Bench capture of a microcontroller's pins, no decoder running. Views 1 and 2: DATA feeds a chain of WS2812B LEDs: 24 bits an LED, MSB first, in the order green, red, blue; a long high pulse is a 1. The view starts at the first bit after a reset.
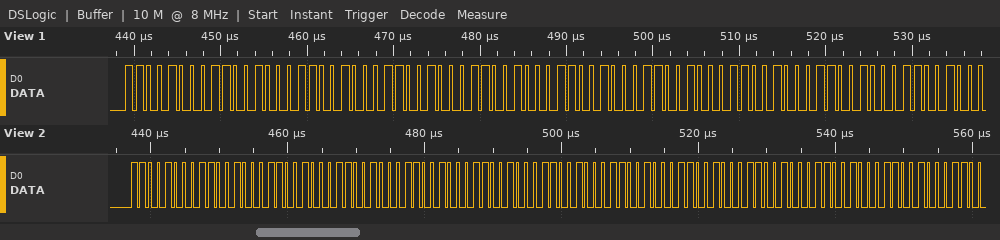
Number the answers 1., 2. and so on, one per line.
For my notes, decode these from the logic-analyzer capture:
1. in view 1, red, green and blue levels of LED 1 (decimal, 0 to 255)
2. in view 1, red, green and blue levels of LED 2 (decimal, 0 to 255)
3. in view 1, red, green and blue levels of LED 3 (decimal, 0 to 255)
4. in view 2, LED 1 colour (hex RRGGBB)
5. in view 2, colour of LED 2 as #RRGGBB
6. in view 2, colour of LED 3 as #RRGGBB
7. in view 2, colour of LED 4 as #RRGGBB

1. 200, 200, 200
2. 200, 200, 200
3. 200, 200, 200
4. #C8C8C8
5. #C8C8C8
6. #C8C8C8
7. #C8C8C8
